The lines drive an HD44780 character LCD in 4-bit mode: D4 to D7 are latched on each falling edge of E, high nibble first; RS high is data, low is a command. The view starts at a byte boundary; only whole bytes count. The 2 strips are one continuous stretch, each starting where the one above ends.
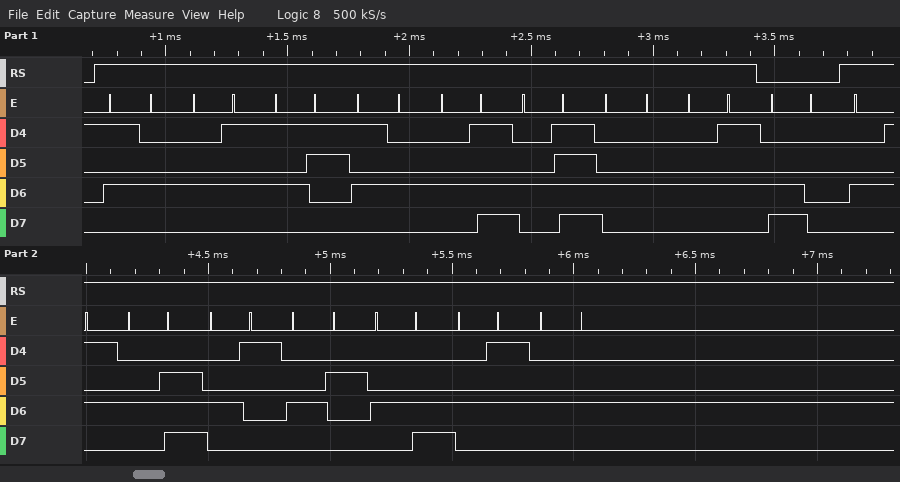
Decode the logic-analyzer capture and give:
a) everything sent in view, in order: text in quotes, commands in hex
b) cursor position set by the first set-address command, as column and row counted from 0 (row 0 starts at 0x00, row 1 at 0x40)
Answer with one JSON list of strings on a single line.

["\"TESTMODE\" 0xC0 \"ENABLED\"", "column 0, row 1"]
